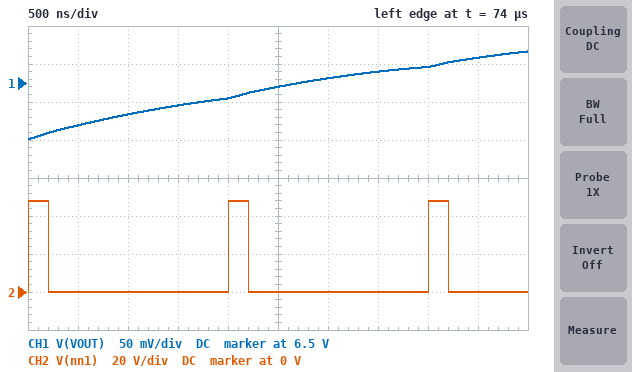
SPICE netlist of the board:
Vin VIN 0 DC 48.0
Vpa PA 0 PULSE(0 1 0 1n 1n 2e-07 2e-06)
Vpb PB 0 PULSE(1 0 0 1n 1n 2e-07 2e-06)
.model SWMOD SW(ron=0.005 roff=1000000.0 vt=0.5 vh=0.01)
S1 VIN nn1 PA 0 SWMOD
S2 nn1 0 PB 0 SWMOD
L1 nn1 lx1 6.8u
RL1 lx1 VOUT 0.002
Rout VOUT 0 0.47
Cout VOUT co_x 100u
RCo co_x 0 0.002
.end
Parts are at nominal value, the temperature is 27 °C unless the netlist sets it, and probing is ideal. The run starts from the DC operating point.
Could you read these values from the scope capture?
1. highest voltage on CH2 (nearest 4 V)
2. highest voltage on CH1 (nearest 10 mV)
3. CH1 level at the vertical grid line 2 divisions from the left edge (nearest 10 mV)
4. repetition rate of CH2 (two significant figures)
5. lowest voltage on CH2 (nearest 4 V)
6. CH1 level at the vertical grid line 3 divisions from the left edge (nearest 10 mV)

48 V
6.54 V
6.46 V
500 kHz
0 V
6.47 V
